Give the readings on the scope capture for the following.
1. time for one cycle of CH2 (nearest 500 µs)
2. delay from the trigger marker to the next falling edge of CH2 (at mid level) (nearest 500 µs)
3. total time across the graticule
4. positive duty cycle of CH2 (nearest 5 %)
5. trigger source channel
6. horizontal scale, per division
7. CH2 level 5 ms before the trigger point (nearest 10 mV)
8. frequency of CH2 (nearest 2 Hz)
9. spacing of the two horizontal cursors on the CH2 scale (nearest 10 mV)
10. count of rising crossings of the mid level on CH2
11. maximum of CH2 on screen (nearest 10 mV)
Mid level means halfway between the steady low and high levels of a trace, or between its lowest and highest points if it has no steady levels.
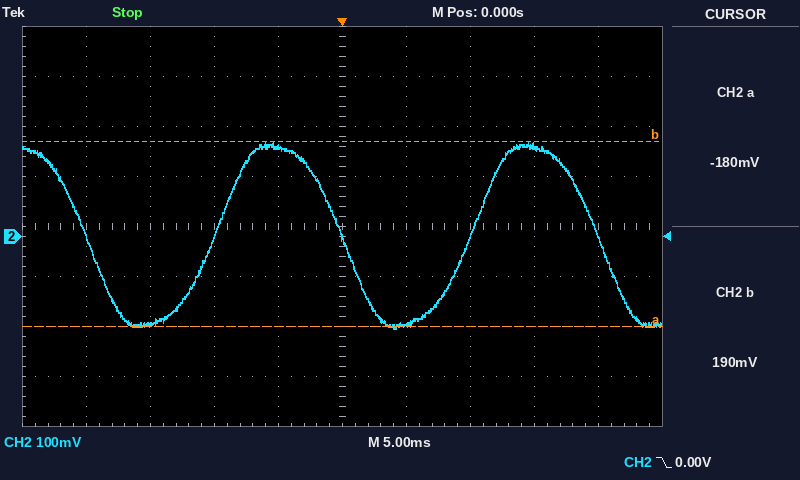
20.0 ms
20.0 ms
50 ms
50 %
CH2
5 ms
180 mV
50 Hz
370 mV
2
190 mV
